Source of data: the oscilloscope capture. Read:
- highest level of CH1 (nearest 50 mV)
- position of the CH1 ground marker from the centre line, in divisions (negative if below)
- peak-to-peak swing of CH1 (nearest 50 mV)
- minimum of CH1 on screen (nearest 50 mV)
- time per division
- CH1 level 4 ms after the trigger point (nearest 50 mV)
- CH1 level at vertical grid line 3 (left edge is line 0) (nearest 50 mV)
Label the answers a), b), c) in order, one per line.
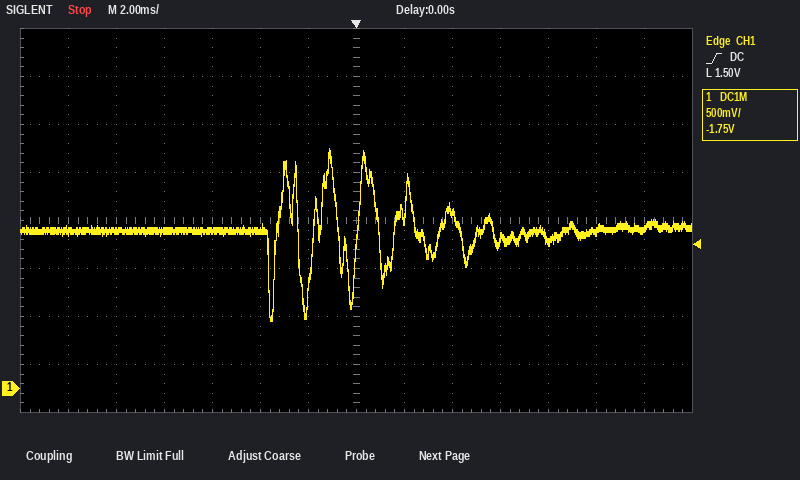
a) 2.50 V
b) -3.5 div
c) 1.80 V
d) 700 mV
e) 2 ms
f) 1.85 V
g) 1.65 V
